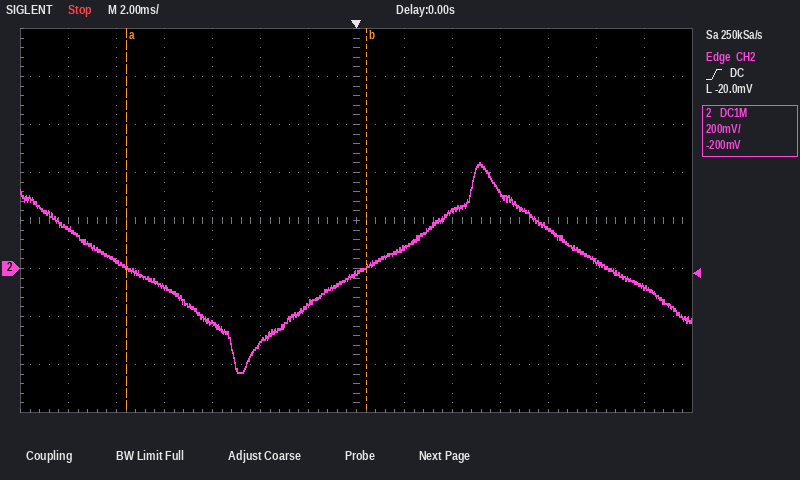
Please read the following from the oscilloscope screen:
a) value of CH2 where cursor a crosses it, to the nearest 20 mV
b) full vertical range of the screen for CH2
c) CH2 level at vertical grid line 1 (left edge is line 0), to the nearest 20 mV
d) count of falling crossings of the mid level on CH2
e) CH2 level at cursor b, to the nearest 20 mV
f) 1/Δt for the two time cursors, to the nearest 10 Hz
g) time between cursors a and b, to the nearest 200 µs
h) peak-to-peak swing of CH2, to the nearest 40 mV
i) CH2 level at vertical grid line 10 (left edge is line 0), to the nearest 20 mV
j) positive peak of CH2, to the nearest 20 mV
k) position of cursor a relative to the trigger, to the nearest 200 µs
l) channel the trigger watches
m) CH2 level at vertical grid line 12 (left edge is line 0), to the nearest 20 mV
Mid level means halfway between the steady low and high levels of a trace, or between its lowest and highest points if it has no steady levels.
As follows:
0 mV
1.6 V
160 mV
2
0 mV
100 Hz
10.0 ms
880 mV
320 mV
440 mV
-9.6 ms
CH2
20 mV
